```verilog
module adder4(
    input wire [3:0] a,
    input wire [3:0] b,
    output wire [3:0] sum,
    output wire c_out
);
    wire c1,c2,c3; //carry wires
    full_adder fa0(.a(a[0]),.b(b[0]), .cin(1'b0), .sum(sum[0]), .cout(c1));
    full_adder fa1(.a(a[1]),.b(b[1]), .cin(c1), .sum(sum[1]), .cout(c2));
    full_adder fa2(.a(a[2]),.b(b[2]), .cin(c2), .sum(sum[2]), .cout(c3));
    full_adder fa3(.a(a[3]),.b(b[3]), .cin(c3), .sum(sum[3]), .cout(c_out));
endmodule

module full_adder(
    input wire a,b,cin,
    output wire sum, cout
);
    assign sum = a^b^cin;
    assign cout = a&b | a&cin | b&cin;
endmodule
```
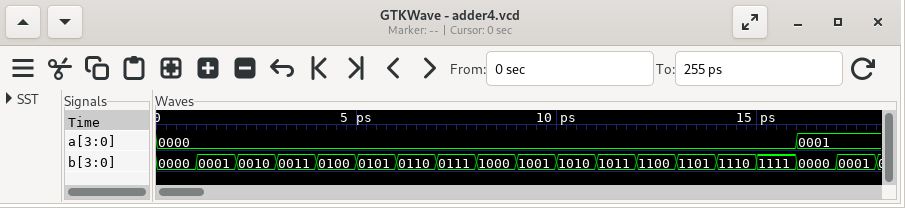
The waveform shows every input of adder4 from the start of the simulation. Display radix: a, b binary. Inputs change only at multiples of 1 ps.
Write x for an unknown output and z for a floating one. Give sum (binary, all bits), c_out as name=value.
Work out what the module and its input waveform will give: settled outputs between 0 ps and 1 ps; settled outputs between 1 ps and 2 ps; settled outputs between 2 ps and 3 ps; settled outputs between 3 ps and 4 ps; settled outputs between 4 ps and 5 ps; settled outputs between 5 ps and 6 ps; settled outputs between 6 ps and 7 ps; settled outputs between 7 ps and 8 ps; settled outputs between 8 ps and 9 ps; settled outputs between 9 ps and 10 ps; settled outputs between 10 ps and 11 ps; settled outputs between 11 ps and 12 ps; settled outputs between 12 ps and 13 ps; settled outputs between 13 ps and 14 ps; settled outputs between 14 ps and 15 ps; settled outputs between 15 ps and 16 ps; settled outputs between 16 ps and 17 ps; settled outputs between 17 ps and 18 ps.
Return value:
sum=0000, c_out=0
sum=0001, c_out=0
sum=0010, c_out=0
sum=0011, c_out=0
sum=0100, c_out=0
sum=0101, c_out=0
sum=0110, c_out=0
sum=0111, c_out=0
sum=1000, c_out=0
sum=1001, c_out=0
sum=1010, c_out=0
sum=1011, c_out=0
sum=1100, c_out=0
sum=1101, c_out=0
sum=1110, c_out=0
sum=1111, c_out=0
sum=0001, c_out=0
sum=0010, c_out=0
